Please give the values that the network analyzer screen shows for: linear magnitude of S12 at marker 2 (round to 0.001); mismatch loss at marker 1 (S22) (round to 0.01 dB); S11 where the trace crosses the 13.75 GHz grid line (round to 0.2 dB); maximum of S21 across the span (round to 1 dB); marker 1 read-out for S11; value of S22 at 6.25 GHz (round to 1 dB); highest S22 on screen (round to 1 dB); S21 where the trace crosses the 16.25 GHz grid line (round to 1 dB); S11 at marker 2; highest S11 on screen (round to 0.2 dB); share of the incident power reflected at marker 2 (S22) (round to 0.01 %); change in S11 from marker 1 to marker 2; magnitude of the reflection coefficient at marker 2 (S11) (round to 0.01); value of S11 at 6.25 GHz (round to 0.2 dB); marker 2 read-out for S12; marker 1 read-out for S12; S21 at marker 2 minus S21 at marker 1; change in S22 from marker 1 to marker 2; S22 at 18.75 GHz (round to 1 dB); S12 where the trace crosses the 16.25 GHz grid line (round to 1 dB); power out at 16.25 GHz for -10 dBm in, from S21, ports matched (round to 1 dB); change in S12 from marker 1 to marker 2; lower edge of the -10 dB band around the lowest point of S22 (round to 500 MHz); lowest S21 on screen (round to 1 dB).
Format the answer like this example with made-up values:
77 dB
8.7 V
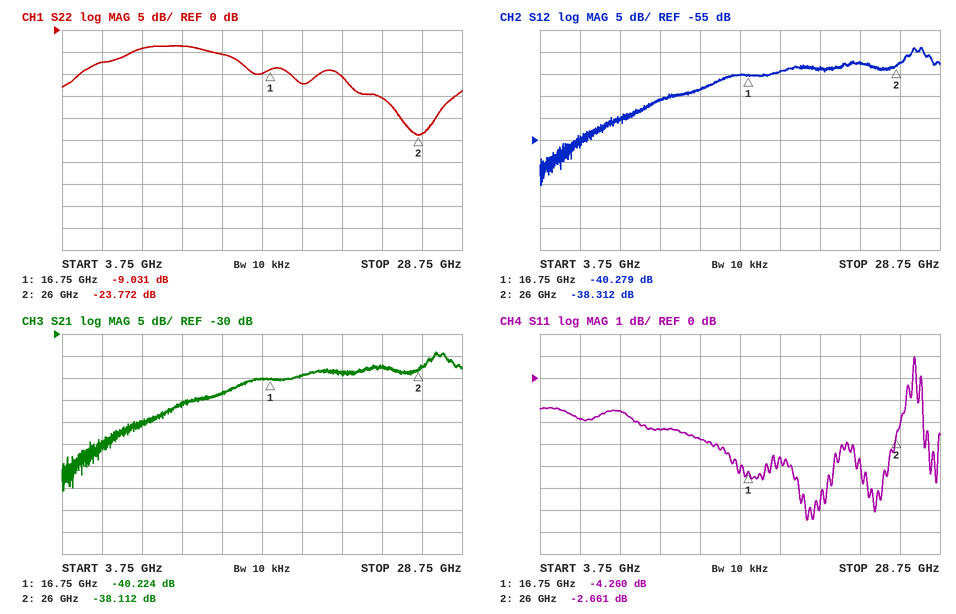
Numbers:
0.012
0.58 dB
-2.8 dB
-34 dB
-4.260 dB
-7 dB
-4 dB
-40 dB
-2.661 dB
1.0 dB
0.42 %
1.599 dB
0.74
-1.8 dB
-38.312 dB
-40.279 dB
2.112 dB
-14.741 dB
-12 dB
-40 dB
-50 dBm
1.967 dB
21.0 GHz
-66 dB
